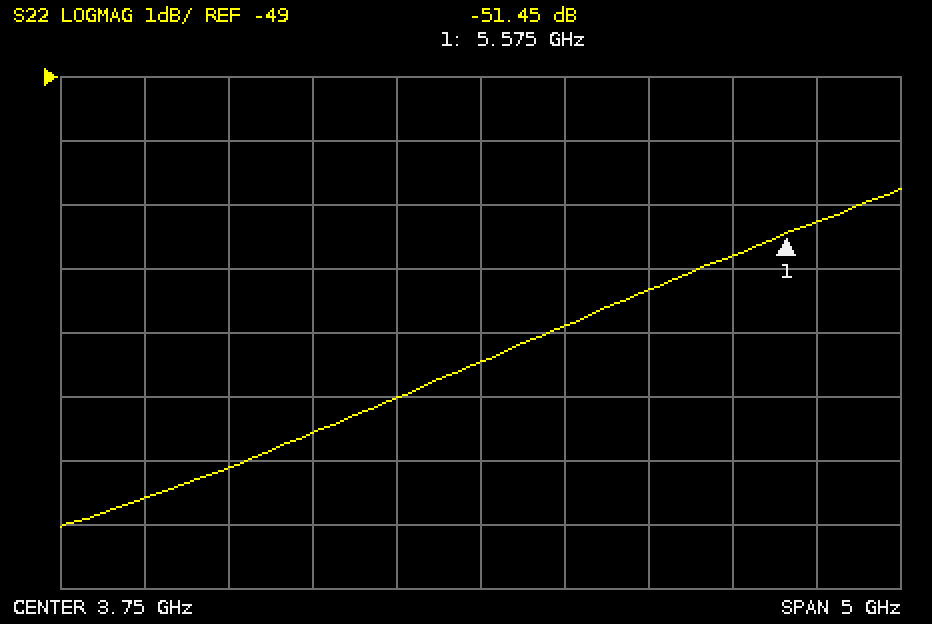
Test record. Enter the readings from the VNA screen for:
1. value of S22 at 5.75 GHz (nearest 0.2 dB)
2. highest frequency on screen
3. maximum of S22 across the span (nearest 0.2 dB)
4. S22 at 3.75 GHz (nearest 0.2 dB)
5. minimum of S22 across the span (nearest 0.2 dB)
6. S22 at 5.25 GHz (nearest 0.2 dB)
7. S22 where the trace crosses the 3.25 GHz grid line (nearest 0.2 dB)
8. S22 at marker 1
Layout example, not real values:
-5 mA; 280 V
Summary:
-51.2 dB; 6.25 GHz; -50.8 dB; -53.4 dB; -56.0 dB; -51.8 dB; -54.0 dB; -51.45 dB
